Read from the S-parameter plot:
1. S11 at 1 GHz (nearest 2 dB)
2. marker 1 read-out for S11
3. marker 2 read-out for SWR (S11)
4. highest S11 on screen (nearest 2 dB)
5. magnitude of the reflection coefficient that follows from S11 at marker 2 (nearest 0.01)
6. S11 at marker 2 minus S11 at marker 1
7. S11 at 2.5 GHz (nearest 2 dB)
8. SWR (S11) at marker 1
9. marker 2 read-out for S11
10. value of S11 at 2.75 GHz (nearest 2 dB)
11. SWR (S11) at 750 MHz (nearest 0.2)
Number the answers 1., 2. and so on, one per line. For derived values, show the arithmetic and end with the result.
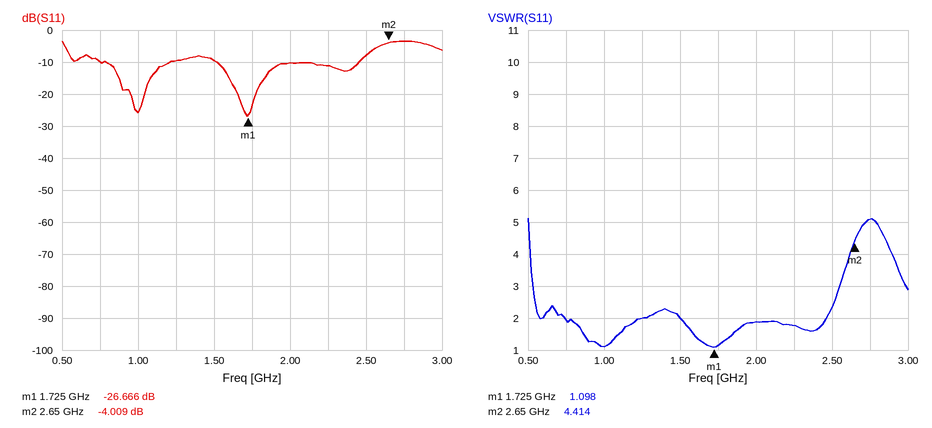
1. -26 dB
2. -26.666 dB
3. 4.414
4. -4 dB
5. 10^(-4.009/20) ≈ 0.63
6. -4.009 − (-26.666) = 22.657 dB
7. -8 dB
8. 1.098
9. -4.009 dB
10. -4 dB
11. 2.0
